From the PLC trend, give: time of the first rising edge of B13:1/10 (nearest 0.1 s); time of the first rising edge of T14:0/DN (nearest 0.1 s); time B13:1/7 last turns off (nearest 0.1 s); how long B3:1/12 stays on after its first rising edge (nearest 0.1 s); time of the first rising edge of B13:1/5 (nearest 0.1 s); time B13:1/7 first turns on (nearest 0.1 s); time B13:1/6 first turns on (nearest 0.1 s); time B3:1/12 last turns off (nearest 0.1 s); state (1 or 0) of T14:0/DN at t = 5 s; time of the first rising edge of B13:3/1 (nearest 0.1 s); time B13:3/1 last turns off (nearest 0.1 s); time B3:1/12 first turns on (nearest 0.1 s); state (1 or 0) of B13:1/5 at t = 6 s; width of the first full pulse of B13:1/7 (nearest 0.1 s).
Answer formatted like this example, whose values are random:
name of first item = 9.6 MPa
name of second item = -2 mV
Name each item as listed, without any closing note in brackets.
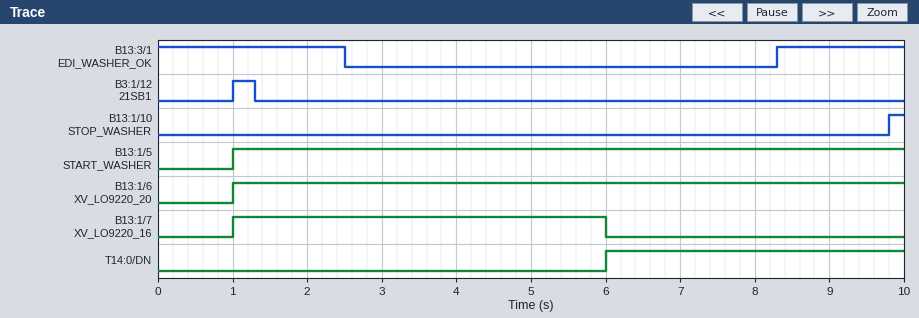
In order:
time of the first rising edge of B13:1/10 = 9.8 s
time of the first rising edge of T14:0/DN = 6.0 s
time B13:1/7 last turns off = 6.0 s
how long B3:1/12 stays on after its first rising edge = 0.3 s
time of the first rising edge of B13:1/5 = 1.0 s
time B13:1/7 first turns on = 1.0 s
time B13:1/6 first turns on = 1.0 s
time B3:1/12 last turns off = 1.3 s
state (1 or 0) of T14:0/DN at t = 5 s = 0
time of the first rising edge of B13:3/1 = 8.3 s
time B13:3/1 last turns off = 2.5 s
time B3:1/12 first turns on = 1.0 s
state (1 or 0) of B13:1/5 at t = 6 s = 1
width of the first full pulse of B13:1/7 = 5.0 s
